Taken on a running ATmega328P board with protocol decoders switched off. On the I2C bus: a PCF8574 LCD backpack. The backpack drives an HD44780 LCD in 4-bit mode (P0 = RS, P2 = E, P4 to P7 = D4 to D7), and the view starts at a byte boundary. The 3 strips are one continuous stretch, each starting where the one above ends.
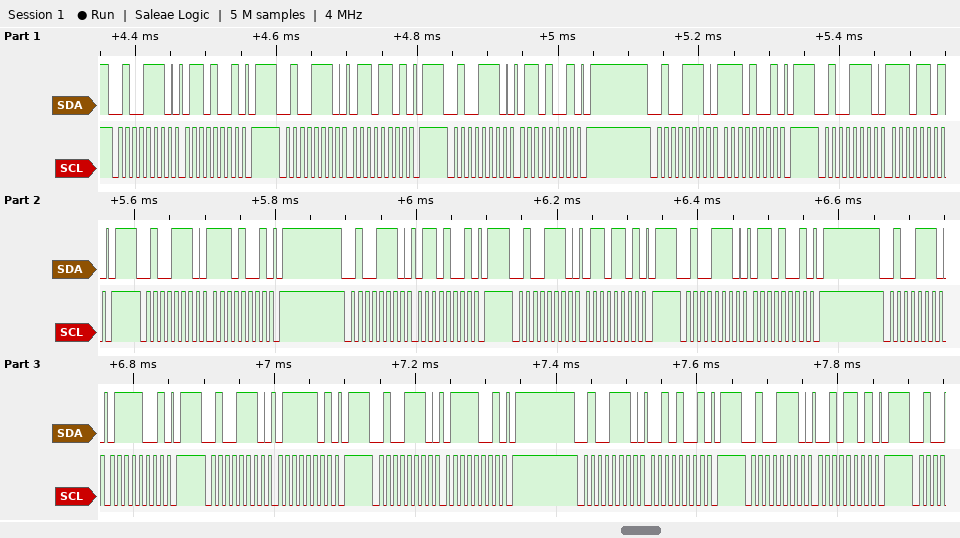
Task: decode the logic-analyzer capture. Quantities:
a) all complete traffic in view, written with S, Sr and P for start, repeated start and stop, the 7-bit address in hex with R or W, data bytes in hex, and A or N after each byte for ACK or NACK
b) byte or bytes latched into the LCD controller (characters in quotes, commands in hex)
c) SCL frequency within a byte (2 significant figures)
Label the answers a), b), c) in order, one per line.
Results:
a) S 27W A 69 A P S 27W A 6D A P S 27W A 69 A P S 27W A E9 A P S 27W A ED A P S 27W A E9 A P S 27W A 69 A P S 27W A 6D A P S 27W A 69 A P S 27W A 79 A P S 27W A 7D A P S 27W A 79 A P S 27W A 29 A P S 27W A 2D A P
b) 'n' 'g'
c) 100 kHz
